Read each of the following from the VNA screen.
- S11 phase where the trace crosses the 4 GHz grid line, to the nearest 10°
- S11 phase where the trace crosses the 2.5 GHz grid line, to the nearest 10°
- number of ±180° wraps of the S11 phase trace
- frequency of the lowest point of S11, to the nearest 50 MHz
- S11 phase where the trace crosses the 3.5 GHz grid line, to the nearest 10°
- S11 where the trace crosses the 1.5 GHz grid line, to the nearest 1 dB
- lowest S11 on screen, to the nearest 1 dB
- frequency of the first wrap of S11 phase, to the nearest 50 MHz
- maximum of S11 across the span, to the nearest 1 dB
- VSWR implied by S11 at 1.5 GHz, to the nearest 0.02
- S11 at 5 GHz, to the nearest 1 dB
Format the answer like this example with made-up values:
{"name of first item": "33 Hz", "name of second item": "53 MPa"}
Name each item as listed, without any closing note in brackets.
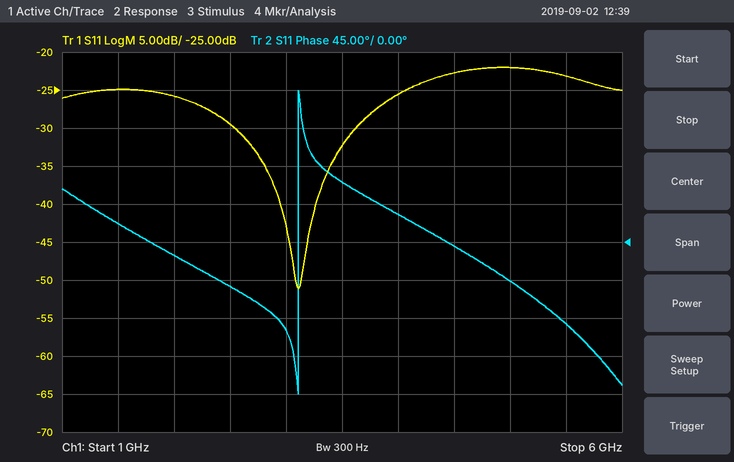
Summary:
{"S11 phase where the trace crosses the 4 GHz grid line, to the nearest 10°": "30°", "S11 phase where the trace crosses the 2.5 GHz grid line, to the nearest 10°": "-50°", "number of ±180° wraps of the S11 phase trace": "1", "frequency of the lowest point of S11, to the nearest 50 MHz": "3.10 GHz", "S11 phase where the trace crosses the 3.5 GHz grid line, to the nearest 10°": "70°", "S11 where the trace crosses the 1.5 GHz grid line, to the nearest 1 dB": "-25 dB", "lowest S11 on screen, to the nearest 1 dB": "-51 dB", "frequency of the first wrap of S11 phase, to the nearest 50 MHz": "3.10 GHz", "maximum of S11 across the span, to the nearest 1 dB": "-22 dB", "VSWR implied by S11 at 1.5 GHz, to the nearest 0.02": "1.12", "S11 at 5 GHz, to the nearest 1 dB": "-22 dB"}
